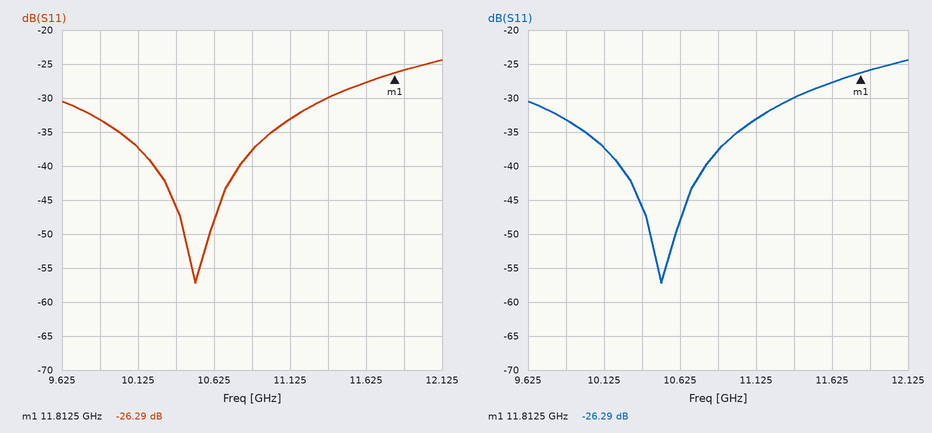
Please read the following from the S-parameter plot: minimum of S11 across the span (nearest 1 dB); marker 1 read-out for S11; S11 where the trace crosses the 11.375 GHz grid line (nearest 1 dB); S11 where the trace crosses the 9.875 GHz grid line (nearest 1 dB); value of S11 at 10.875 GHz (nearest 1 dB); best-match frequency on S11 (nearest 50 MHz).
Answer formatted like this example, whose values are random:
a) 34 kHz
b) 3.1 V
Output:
a) -57 dB
b) -26.29 dB
c) -30 dB
d) -33 dB
e) -38 dB
f) 10.50 GHz
